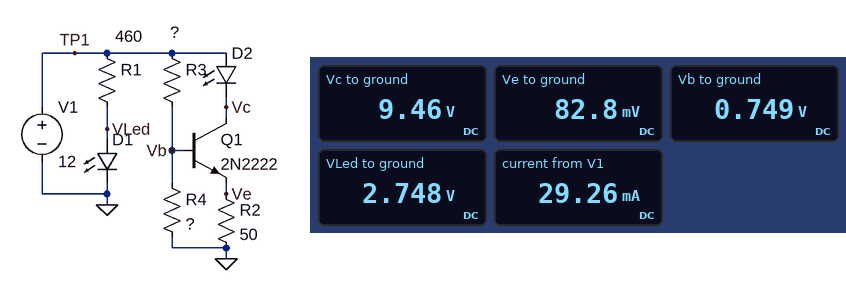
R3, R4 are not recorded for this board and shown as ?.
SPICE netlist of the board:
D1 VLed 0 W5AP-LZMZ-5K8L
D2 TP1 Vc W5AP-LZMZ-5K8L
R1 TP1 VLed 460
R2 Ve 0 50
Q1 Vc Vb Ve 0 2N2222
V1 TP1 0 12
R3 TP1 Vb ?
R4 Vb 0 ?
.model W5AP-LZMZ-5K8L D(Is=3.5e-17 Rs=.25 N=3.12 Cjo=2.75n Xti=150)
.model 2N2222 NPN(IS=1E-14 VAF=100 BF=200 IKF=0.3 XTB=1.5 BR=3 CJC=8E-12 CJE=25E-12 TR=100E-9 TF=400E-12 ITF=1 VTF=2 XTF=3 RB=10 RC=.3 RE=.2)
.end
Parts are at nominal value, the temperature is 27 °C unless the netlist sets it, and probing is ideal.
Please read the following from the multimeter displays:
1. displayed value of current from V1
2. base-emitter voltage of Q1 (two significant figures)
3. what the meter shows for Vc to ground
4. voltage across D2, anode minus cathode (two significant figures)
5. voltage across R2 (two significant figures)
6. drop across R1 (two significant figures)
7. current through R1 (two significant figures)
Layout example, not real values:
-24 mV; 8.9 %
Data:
29.26 mA; 670 mV; 9.46 V; 2.5 V; 83 mV; 9.3 V; 20 mA
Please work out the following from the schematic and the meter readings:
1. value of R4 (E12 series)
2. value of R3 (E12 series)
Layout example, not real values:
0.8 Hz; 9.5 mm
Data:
100 Ω; 1.5 kΩ
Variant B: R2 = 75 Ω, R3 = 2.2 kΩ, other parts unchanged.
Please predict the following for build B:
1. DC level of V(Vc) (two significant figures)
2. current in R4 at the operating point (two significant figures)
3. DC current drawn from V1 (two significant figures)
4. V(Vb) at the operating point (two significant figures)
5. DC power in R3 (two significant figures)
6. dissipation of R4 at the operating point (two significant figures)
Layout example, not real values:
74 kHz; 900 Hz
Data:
9.9 V; 5.2 mA; 25 mA; 520 mV; 60 mW; 2.7 mW
